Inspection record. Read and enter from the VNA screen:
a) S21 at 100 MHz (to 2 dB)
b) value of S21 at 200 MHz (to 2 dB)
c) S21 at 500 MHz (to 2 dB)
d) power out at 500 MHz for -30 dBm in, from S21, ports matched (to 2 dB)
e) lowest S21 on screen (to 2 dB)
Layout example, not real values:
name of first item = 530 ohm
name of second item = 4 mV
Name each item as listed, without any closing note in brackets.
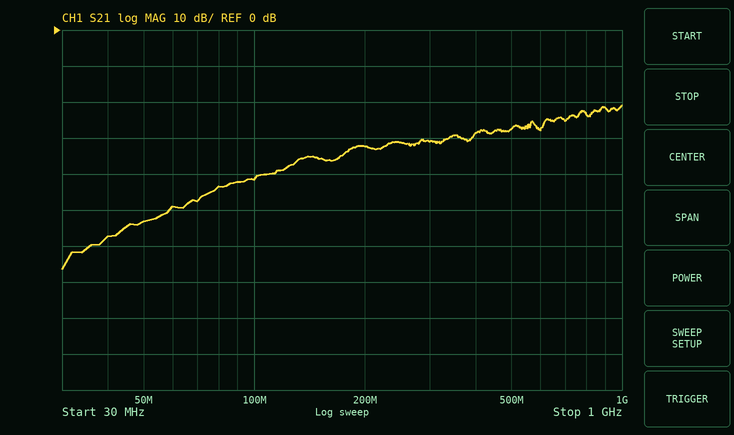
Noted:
S21 at 100 MHz = -42 dB
value of S21 at 200 MHz = -32 dB
S21 at 500 MHz = -28 dB
power out at 500 MHz for -30 dBm in, from S21, ports matched = -58 dBm
lowest S21 on screen = -66 dB
